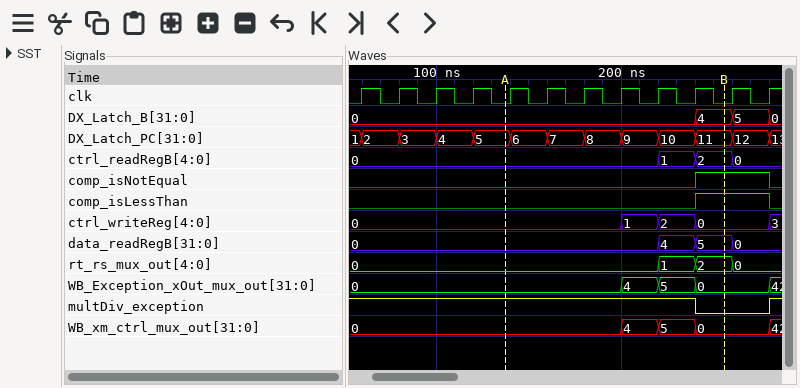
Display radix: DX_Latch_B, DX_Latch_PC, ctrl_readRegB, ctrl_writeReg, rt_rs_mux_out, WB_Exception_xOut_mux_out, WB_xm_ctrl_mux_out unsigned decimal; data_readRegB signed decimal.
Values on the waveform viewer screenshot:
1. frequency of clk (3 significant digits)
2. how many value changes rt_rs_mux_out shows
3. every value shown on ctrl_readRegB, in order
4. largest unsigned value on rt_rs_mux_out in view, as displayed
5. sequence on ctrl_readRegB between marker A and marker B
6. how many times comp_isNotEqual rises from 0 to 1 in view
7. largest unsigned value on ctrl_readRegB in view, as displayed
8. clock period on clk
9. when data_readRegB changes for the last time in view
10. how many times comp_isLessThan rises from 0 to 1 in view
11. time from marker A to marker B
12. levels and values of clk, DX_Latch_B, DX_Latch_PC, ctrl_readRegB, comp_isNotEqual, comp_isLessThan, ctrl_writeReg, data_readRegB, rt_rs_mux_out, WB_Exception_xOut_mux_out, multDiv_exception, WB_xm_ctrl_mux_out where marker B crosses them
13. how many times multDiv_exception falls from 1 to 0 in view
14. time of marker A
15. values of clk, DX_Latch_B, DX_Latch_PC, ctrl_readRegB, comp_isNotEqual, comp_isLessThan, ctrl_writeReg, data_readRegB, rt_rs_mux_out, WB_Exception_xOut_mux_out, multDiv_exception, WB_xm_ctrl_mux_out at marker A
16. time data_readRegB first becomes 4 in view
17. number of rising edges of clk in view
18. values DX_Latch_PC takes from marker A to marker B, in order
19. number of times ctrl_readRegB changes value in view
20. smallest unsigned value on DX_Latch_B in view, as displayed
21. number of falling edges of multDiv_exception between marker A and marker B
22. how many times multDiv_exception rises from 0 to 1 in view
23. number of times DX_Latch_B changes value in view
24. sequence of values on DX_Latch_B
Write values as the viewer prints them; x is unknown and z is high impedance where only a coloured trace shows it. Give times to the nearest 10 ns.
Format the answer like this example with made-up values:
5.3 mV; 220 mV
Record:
50.0 MHz; 3; 0, 1, 2, 0; 2; 0, 1, 2; 1; 2; 20 ns; 260 ns; 1; 120 ns; clk=0, DX_Latch_B=4, DX_Latch_PC=11, ctrl_readRegB=2, comp_isNotEqual=1, comp_isLessThan=1, ctrl_writeReg=0, data_readRegB=5, rt_rs_mux_out=2, WB_Exception_xOut_mux_out=0, multDiv_exception=0, WB_xm_ctrl_mux_out=0; 1; 140 ns; clk=0, DX_Latch_B=0, DX_Latch_PC=5, ctrl_readRegB=0, comp_isNotEqual=0, comp_isLessThan=0, ctrl_writeReg=0, data_readRegB=0, rt_rs_mux_out=0, WB_Exception_xOut_mux_out=0, multDiv_exception=1, WB_xm_ctrl_mux_out=0; 220 ns; 12; 5, 6, 7, 8, 9, 10, 11; 3; 0; 1; 1; 3; 0, 4, 5, 0
